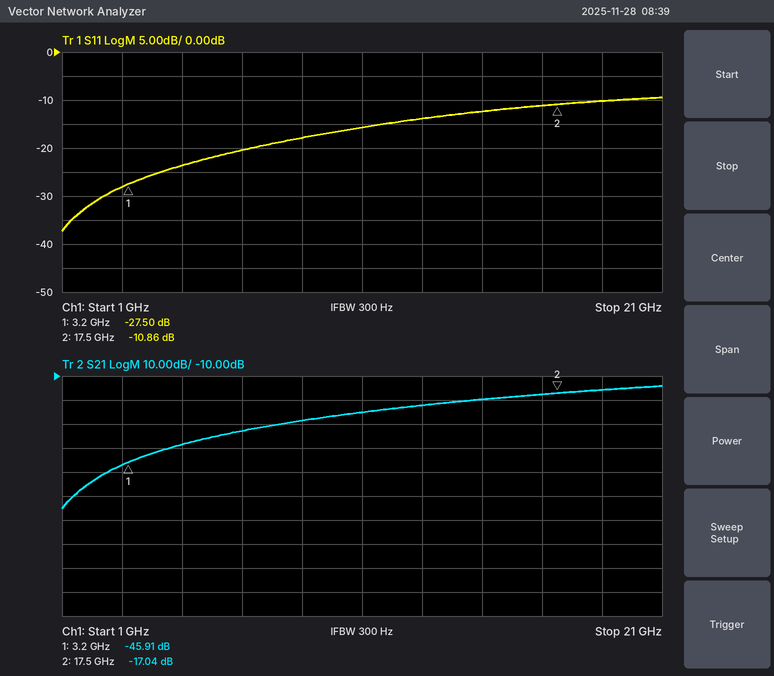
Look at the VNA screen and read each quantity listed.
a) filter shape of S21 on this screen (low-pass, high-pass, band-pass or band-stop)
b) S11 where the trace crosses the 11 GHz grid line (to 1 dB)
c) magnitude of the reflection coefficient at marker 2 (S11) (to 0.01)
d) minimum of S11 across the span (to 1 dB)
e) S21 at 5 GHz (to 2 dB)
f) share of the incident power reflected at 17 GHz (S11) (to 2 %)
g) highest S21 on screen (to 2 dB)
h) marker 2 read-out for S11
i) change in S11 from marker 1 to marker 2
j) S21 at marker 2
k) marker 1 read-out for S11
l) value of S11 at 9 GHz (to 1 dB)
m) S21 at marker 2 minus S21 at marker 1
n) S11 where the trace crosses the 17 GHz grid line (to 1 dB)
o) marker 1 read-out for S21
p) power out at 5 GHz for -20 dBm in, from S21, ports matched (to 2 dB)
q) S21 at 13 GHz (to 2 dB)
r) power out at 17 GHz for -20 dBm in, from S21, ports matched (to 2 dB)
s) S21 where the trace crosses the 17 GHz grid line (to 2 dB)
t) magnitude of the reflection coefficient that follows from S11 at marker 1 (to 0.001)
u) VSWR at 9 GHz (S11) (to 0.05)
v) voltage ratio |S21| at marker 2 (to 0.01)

high-pass
-16 dB
0.29
-37 dB
-38 dB
8 %
-14 dB
-10.86 dB
16.64 dB
-17.04 dB
-27.50 dB
-18 dB
28.87 dB
-11 dB
-45.91 dB
-58 dBm
-22 dB
-38 dBm
-18 dB
0.042
1.30
0.14
